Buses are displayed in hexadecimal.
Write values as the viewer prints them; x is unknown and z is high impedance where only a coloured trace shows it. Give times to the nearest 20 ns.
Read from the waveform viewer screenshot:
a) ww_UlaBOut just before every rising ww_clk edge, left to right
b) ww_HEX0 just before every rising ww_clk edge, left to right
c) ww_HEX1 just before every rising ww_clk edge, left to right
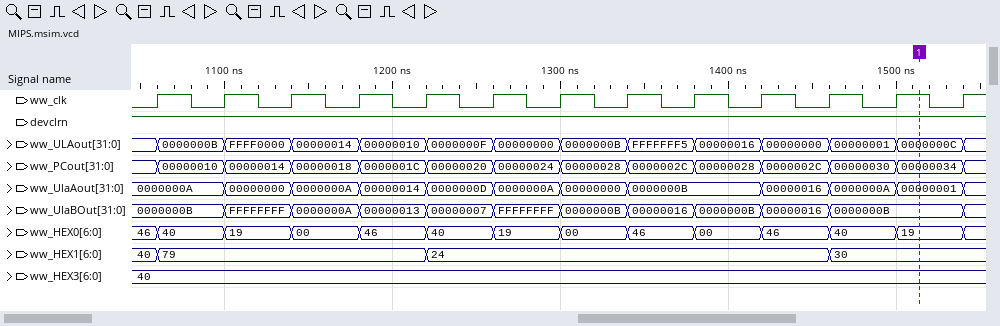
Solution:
0000000B, 0000000B, FFFFFFFF, 0000000A, 00000013, 00000007, FFFFFFFF, 0000000B, 00000016, 0000000B, 00000016, 0000000B, 0000000B
46, 40, 19, 00, 46, 40, 19, 00, 46, 00, 46, 40, 19
40, 79, 79, 79, 79, 24, 24, 24, 24, 24, 24, 30, 30
